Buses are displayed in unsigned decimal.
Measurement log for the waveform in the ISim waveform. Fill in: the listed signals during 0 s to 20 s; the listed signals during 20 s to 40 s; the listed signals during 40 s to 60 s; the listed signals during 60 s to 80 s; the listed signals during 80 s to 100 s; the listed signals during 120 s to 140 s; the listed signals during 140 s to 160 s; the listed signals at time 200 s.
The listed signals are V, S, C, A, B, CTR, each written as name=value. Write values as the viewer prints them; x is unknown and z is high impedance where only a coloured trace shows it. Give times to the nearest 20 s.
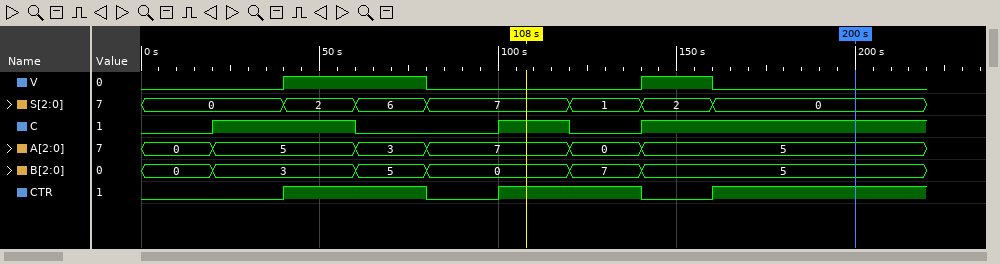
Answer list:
V=0, S=0, C=0, A=0, B=0, CTR=0
V=0, S=0, C=1, A=5, B=3, CTR=0
V=1, S=2, C=1, A=5, B=3, CTR=1
V=1, S=6, C=0, A=3, B=5, CTR=1
V=0, S=7, C=0, A=7, B=0, CTR=0
V=0, S=1, C=0, A=0, B=7, CTR=1
V=1, S=2, C=1, A=5, B=5, CTR=0
V=0, S=0, C=1, A=5, B=5, CTR=1
